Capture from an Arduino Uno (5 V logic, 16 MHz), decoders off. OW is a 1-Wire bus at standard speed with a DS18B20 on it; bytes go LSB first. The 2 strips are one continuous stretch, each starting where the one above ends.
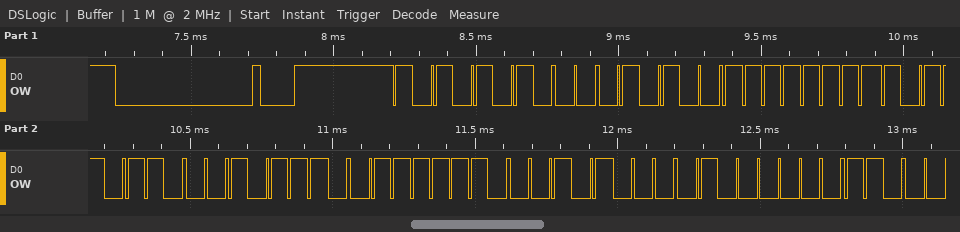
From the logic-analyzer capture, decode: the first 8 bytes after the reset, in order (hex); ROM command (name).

55 28 FF 6D 74 7E 14 02
Match ROM
